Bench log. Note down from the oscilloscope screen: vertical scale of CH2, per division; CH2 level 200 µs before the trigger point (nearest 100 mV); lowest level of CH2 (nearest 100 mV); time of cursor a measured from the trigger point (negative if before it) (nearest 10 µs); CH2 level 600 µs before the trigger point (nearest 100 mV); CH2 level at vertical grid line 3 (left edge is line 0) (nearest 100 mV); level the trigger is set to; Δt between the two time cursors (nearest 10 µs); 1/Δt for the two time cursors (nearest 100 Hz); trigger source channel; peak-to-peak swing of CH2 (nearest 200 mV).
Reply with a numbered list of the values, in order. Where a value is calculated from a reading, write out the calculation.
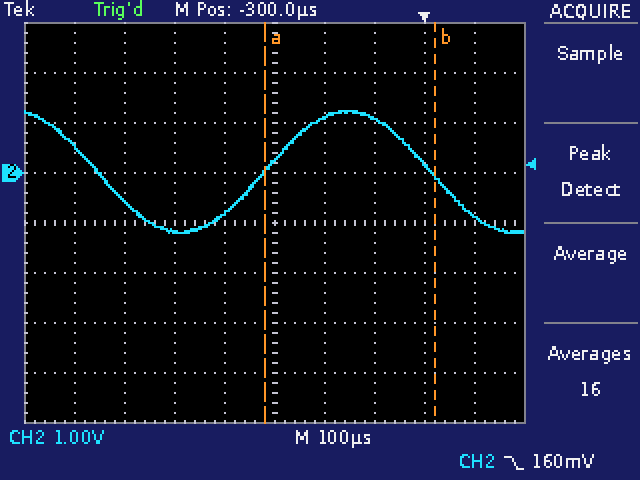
1. 1 V
2. 1.1 V
3. -1.2 V
4. -320 µs
5. -600 mV
6. -1.2 V
7. 160 mV
8. 340 µs
9. 1 / 340 µs ≈ 2.9 kHz
10. CH2
11. 2.4 V
